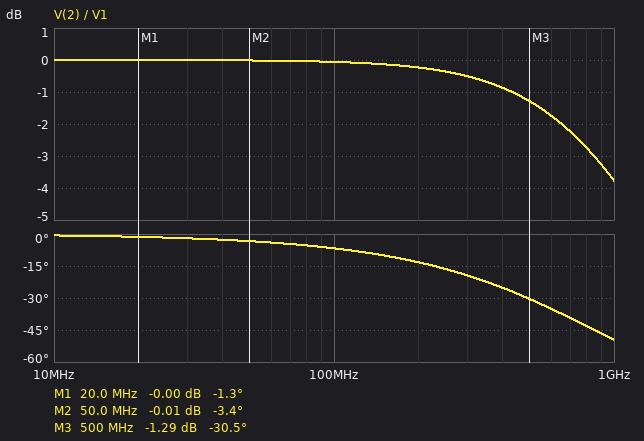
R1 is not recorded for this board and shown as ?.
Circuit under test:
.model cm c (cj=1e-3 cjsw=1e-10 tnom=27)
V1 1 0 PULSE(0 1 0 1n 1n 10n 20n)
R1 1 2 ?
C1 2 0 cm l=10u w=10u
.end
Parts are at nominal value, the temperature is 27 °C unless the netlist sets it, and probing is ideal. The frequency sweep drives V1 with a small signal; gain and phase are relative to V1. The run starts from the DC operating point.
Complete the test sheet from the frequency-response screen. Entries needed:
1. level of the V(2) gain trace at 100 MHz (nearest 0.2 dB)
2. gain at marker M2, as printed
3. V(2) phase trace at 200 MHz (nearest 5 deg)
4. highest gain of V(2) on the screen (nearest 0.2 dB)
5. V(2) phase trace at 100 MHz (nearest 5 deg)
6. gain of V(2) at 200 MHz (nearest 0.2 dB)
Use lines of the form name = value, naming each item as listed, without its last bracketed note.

level of the V(2) gain trace at 100 MHz = 0 dB
gain at marker M2, as printed = -0.01 dB
V(2) phase trace at 200 MHz = -15 deg
highest gain of V(2) on the screen = 0 dB
V(2) phase trace at 100 MHz = -5 deg
gain of V(2) at 200 MHz = -0.2 dB
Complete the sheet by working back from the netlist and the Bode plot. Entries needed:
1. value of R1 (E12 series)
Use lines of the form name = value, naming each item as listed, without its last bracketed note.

value of R1 = 1.8 kΩ
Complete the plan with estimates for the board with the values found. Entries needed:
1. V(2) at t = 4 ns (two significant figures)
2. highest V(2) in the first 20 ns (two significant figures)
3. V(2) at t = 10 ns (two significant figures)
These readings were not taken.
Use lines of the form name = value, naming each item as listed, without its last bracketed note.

V(2) at t = 4 ns = 1.0 V
highest V(2) in the first 20 ns = 1.0 V
V(2) at t = 10 ns = 1.0 V
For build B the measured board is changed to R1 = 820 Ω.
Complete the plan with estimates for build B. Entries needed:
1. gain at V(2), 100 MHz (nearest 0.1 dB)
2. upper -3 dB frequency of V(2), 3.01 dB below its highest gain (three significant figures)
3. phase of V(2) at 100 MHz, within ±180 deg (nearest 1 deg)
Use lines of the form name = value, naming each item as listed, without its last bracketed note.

gain at V(2), 100 MHz = 0 dB
upper -3 dB frequency of V(2), 3.01 dB below its highest gain = 1.87 GHz
phase of V(2) at 100 MHz, within ±180 deg = -3 deg
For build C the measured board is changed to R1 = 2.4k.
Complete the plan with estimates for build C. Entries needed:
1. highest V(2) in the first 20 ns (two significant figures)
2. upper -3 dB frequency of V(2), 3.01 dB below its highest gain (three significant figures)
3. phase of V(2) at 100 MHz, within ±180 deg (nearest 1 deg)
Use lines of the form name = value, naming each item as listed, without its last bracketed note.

highest V(2) in the first 20 ns = 1.0 V
upper -3 dB frequency of V(2), 3.01 dB below its highest gain = 638 MHz
phase of V(2) at 100 MHz, within ±180 deg = -9 deg
